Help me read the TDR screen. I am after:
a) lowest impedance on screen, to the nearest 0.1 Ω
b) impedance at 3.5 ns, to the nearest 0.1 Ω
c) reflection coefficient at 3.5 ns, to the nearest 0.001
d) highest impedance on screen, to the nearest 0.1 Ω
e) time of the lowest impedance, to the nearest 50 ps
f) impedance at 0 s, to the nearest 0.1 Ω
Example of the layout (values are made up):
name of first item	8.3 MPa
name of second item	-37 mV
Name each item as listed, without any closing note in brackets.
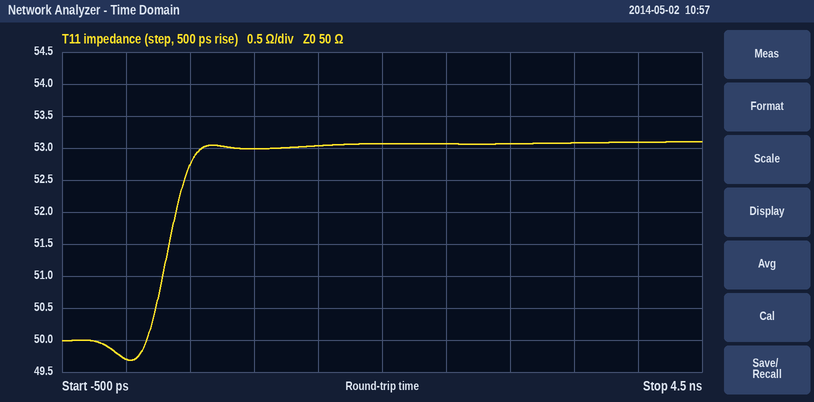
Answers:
lowest impedance on screen, to the nearest 0.1 Ω	49.7 Ω
impedance at 3.5 ns, to the nearest 0.1 Ω	53.1 Ω
reflection coefficient at 3.5 ns, to the nearest 0.001	+0.030
highest impedance on screen, to the nearest 0.1 Ω	53.1 Ω
time of the lowest impedance, to the nearest 50 ps	50 ps
impedance at 0 s, to the nearest 0.1 Ω	49.7 Ω
